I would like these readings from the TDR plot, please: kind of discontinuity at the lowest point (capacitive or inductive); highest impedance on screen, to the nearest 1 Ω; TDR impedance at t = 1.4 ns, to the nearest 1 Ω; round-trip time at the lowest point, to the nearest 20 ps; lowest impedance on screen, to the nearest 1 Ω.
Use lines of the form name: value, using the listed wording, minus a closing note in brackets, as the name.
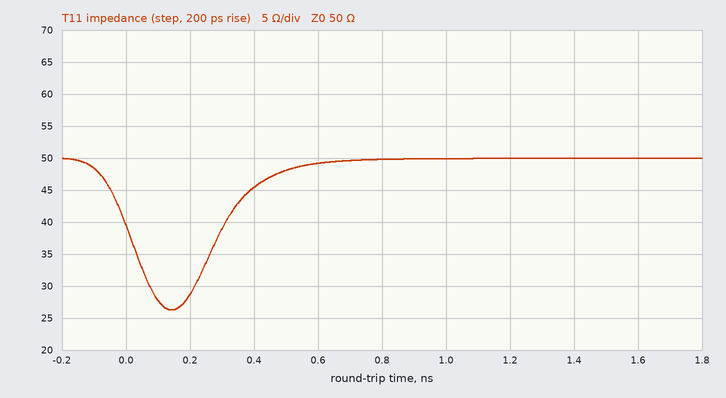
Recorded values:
kind of discontinuity at the lowest point: capacitive
highest impedance on screen, to the nearest 1 Ω: 50 Ω
TDR impedance at t = 1.4 ns, to the nearest 1 Ω: 50 Ω
round-trip time at the lowest point, to the nearest 20 ps: 140 ps
lowest impedance on screen, to the nearest 1 Ω: 26 Ω
